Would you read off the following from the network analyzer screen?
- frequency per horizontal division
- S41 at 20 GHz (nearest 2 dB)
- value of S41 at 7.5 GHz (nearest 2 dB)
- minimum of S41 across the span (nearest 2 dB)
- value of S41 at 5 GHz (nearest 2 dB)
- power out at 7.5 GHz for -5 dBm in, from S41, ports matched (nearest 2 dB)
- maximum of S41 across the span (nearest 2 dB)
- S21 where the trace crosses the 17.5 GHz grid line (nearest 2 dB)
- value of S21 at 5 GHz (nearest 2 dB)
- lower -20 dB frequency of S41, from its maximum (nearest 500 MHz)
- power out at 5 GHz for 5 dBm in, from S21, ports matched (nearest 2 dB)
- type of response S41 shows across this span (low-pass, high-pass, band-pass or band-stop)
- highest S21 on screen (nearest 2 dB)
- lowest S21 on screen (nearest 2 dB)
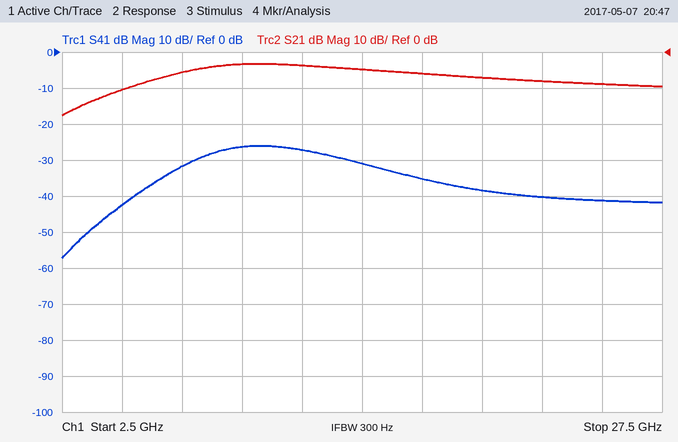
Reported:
2.5 GHz
-38 dB
-32 dB
-58 dB
-42 dB
-36 dBm
-26 dB
-6 dB
-10 dB
4.5 GHz
-6 dBm
band-pass
-4 dB
-18 dB
